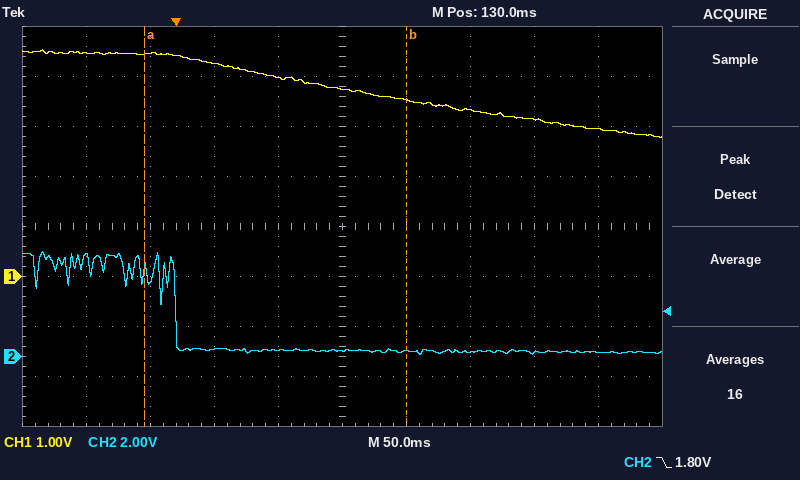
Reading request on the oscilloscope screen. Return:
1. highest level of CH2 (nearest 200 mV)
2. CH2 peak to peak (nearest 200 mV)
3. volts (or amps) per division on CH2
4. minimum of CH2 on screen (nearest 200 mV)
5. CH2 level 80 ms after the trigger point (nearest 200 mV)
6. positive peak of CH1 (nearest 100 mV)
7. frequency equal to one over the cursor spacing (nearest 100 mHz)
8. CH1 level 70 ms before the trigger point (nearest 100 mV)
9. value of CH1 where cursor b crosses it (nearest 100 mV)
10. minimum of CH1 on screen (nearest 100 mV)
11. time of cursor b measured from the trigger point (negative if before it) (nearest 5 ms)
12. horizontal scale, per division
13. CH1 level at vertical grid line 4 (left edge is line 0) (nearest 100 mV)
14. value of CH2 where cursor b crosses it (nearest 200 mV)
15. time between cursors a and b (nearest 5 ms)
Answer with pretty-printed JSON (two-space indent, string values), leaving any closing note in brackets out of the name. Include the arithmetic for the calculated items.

{
  "highest level of CH2": "4.2 V",
  "CH2 peak to peak": "4.2 V − (0.0 V) = 4.2 V",
  "volts (or amps) per division on CH2": "2 V",
  "minimum of CH2 on screen": "0.0 V",
  "CH2 level 80 ms after the trigger point": "200 mV",
  "positive peak of CH1": "4.5 V",
  "frequency equal to one over the cursor spacing": "1 / 205 ms ≈ 4.9 Hz",
  "CH1 level 70 ms before the trigger point": "4.5 V",
  "value of CH1 where cursor b crosses it": "3.5 V",
  "minimum of CH1 on screen": "2.8 V",
  "time of cursor b measured from the trigger point (negative if before it)": "+180 ms",
  "horizontal scale, per division": "50 ms",
  "CH1 level at vertical grid line 4 (left edge is line 0)": "4.0 V",
  "value of CH2 where cursor b crosses it": "200 mV",
  "time between cursors a and b": "205 ms"
}
